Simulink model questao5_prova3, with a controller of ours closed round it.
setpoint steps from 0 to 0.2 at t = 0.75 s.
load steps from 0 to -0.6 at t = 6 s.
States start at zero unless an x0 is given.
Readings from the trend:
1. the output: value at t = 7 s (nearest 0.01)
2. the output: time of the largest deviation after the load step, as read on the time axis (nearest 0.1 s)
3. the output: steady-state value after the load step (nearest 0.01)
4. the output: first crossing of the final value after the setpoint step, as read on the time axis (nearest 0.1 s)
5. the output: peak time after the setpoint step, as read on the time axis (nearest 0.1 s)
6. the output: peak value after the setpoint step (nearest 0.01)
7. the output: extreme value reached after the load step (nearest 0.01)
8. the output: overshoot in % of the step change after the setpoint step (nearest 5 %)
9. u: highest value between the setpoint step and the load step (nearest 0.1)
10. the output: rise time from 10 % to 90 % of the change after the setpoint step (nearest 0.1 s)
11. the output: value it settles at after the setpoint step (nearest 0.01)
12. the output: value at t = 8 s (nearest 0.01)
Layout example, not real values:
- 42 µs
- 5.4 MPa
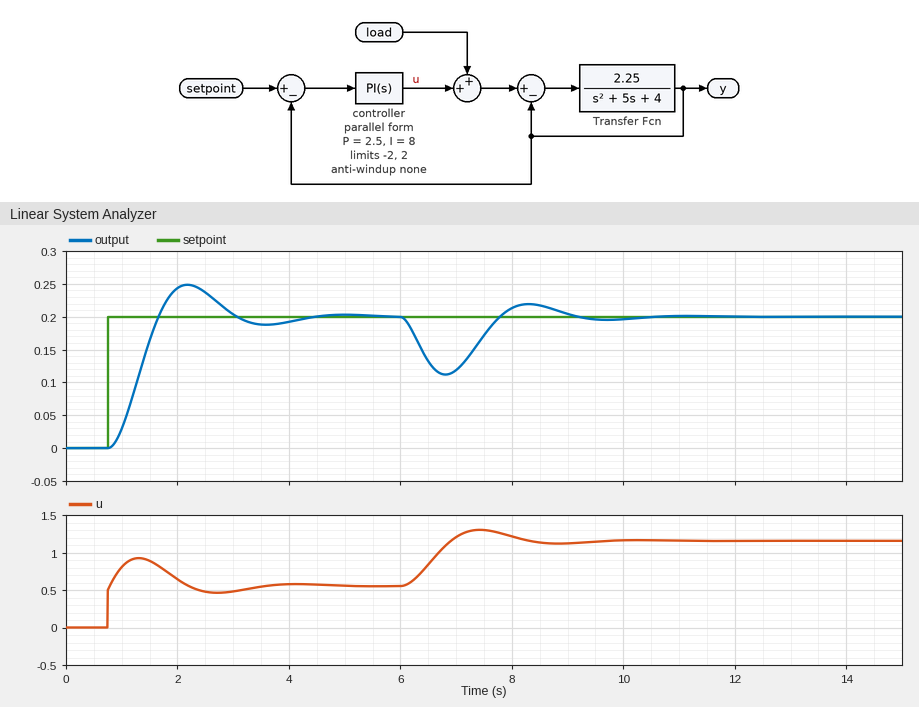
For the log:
- 0.12
- 6.8 s
- 0.20
- 1.7 s
- 2.2 s
- 0.25
- 0.11
- 25 %
- 0.9
- 0.6 s
- 0.20
- 0.21
